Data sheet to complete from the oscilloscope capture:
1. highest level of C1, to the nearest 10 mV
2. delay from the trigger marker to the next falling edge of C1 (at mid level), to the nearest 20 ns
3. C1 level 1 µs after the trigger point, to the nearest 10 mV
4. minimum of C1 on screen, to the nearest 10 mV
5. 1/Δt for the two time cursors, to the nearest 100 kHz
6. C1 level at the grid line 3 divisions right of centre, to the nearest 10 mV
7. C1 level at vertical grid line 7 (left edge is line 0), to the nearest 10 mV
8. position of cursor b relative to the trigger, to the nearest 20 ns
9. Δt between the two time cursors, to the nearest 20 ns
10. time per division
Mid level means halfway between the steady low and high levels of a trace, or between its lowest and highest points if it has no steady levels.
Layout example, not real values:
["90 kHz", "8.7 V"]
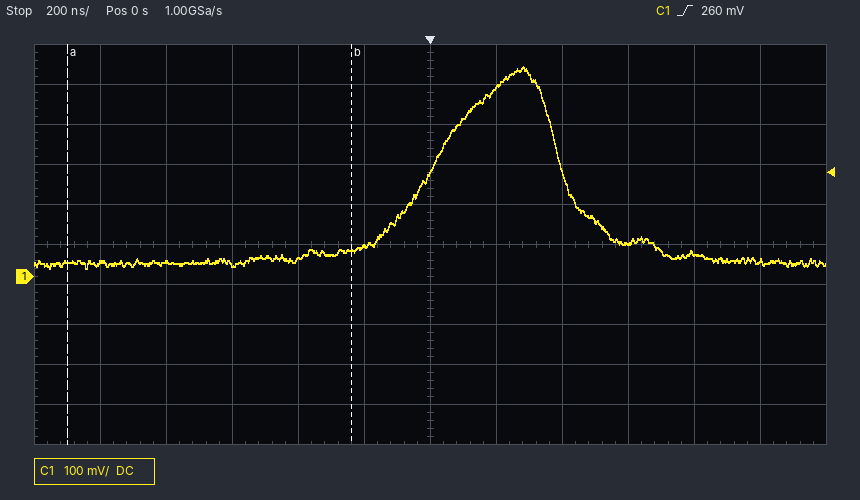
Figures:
["520 mV", "400 ns", "40 mV", "20 mV", "1.2 MHz", "80 mV", "470 mV", "-240 ns", "860 ns", "200 ns"]
